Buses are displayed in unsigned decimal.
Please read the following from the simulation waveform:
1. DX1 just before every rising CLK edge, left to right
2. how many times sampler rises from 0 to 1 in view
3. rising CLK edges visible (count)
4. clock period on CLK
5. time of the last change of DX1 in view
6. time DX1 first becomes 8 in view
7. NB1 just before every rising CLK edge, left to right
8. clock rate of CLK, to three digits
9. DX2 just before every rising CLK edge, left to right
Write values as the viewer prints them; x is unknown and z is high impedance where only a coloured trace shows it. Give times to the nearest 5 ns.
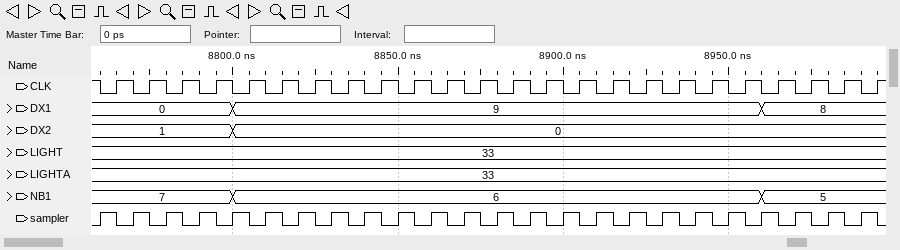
0, 0, 0, 0, 9, 9, 9, 9, 9, 9, 9, 9, 9, 9, 9, 9, 9, 9, 9, 9, 8, 8, 8, 8
24
24
10 ns
8960 ns
8960 ns
7, 7, 7, 7, 6, 6, 6, 6, 6, 6, 6, 6, 6, 6, 6, 6, 6, 6, 6, 6, 5, 5, 5, 5
100 MHz
1, 1, 1, 1, 0, 0, 0, 0, 0, 0, 0, 0, 0, 0, 0, 0, 0, 0, 0, 0, 0, 0, 0, 0
